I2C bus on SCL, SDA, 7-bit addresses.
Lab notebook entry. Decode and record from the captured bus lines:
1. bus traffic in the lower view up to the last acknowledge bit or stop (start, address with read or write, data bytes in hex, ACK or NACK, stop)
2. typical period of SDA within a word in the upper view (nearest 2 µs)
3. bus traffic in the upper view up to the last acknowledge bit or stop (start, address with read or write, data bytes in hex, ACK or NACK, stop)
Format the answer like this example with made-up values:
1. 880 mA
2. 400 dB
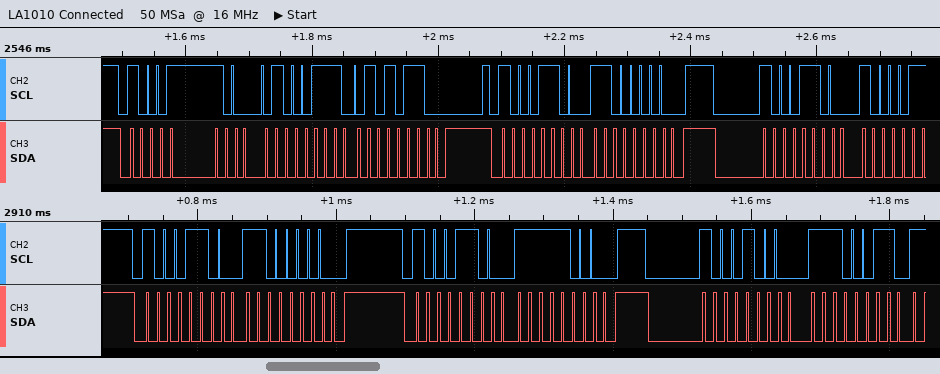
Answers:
1. start, address 46 write ACK, C0 ACK, stop, start, address 46 write ACK, F8 ACK, stop, start, address 44 write ACK, E3 ACK
2. 16 µs
3. start, address 46 write ACK, 47 ACK, 56 ACK, stop, start, address 46 write ACK, C0 ACK, stop, start, address 46 write ACK
